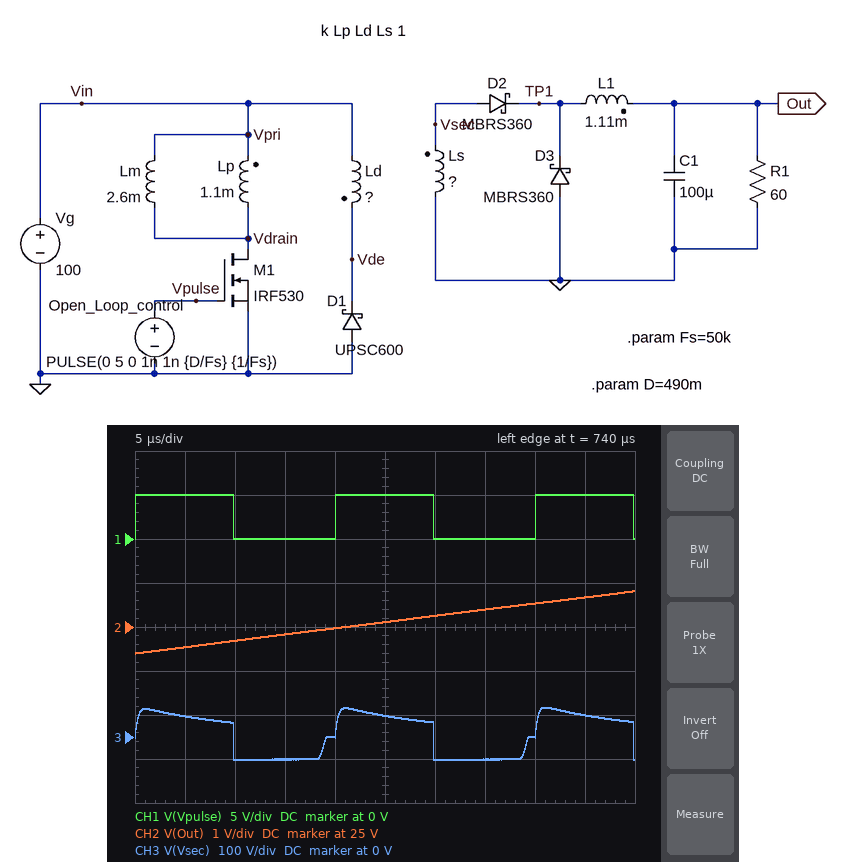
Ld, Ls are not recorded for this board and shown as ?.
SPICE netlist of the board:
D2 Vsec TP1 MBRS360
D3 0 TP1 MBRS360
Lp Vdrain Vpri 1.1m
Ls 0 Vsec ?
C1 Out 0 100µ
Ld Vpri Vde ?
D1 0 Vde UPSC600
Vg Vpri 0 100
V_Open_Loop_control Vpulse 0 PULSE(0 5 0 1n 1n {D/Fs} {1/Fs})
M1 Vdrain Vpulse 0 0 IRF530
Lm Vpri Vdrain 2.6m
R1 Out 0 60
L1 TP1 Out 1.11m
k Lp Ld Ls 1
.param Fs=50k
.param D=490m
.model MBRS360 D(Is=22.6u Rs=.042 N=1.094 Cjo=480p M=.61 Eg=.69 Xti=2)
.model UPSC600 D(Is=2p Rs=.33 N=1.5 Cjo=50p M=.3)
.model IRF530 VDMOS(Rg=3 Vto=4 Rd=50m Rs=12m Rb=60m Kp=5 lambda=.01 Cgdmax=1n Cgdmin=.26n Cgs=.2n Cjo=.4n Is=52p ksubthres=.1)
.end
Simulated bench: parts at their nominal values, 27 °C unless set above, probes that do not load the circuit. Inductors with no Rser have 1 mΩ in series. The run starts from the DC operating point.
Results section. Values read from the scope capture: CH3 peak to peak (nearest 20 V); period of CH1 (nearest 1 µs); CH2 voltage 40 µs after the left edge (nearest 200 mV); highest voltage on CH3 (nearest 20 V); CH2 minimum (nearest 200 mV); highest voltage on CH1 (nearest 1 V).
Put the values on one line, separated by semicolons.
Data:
120 V; 20 µs; 25.6 V; 60 V; 24.4 V; 5 V
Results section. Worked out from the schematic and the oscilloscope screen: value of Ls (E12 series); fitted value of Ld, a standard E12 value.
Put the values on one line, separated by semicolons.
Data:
1 mH; 3.9 mH
